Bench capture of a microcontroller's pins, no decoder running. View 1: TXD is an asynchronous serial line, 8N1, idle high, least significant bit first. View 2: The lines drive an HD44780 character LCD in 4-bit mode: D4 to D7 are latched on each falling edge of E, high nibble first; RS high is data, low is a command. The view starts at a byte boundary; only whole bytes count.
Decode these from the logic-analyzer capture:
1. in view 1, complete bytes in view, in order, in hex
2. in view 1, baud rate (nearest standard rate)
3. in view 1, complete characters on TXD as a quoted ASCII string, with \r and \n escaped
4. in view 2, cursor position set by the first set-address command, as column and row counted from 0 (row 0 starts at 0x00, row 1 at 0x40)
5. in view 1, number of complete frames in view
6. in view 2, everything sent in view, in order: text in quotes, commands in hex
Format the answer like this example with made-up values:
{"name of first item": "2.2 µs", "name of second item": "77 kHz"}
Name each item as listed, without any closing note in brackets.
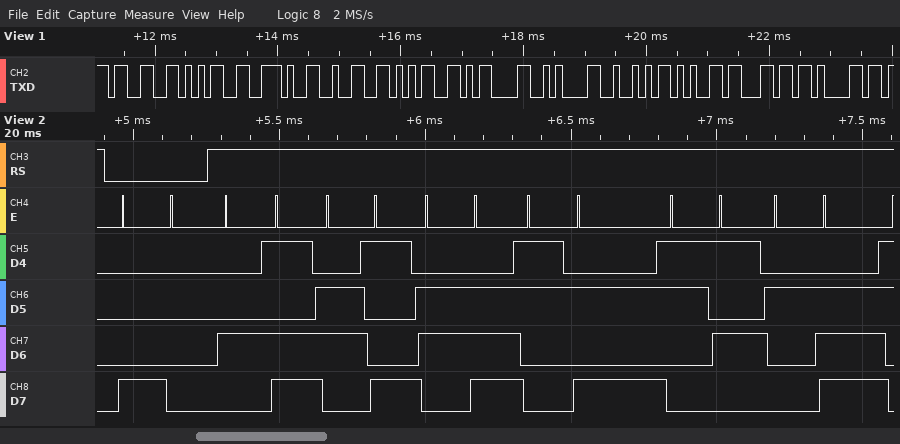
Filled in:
{"in view 1, complete bytes in view, in order, in hex": "0x33 0x35 0x2E 0x32 0x35 0x0D 0x0A 0x52 0x65 0x6C 0x61", "in view 1, baud rate": "9600 baud", "in view 1, complete characters on TXD as a quoted ASCII string, with \\r and \\n escaped": "\"35.25\\r\\nRela\"", "in view 2, cursor position set by the first set-address command, as column and row counted from 0": "column 0, row 0", "in view 1, number of complete frames in view": "11", "in view 2, everything sent in view, in order: text in quotes, commands in hex": "0x80 \"Min:5.\""}
